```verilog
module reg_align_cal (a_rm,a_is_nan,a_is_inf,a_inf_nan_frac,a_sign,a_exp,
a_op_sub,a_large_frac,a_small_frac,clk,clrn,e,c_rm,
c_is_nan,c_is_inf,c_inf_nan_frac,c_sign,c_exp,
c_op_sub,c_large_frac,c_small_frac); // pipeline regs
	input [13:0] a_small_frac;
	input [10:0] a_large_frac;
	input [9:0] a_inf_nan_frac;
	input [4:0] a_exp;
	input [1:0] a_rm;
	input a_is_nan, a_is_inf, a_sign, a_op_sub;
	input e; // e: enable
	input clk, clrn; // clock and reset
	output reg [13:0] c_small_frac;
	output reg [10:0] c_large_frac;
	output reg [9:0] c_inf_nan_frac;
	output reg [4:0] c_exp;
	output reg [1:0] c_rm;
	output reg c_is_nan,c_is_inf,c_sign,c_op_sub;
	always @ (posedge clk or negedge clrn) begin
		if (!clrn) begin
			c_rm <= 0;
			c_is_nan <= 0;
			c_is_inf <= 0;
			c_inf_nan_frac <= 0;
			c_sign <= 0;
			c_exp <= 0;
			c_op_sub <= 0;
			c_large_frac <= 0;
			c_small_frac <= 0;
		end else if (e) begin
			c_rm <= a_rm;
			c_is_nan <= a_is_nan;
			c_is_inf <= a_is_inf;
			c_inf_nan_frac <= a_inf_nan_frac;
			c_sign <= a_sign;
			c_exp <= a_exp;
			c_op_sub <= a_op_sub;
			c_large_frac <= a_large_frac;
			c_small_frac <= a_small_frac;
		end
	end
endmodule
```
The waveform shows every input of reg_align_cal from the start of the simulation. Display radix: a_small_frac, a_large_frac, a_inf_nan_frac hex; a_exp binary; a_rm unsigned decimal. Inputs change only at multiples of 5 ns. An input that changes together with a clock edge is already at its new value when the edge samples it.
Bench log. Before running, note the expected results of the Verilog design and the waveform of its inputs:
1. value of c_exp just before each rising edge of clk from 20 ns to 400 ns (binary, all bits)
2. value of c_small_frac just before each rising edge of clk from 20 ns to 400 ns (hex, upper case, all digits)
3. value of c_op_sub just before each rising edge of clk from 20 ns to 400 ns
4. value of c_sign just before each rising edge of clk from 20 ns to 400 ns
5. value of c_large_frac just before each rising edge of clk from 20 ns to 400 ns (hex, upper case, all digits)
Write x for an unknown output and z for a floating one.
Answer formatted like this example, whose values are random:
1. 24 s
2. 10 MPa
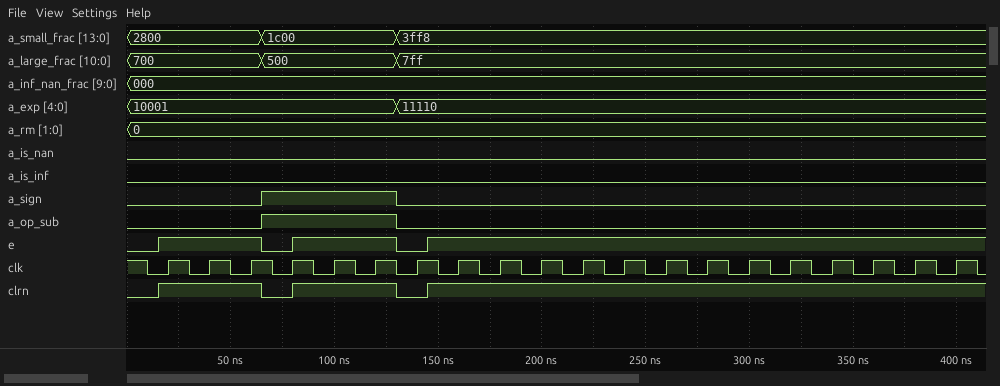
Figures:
1. 00000, 10001, 10001, 00000, 10001, 10001, 00000, 00000, 11110, 11110, 11110, 11110, 11110, 11110, 11110, 11110, 11110, 11110, 11110, 11110
2. 0000, 2800, 2800, 0000, 1C00, 1C00, 0000, 0000, 3FF8, 3FF8, 3FF8, 3FF8, 3FF8, 3FF8, 3FF8, 3FF8, 3FF8, 3FF8, 3FF8, 3FF8
3. 0 0 0 0 1 1 0 0 0 0 0 0 0 0 0 0 0 0 0 0
4. 0 0 0 0 1 1 0 0 0 0 0 0 0 0 0 0 0 0 0 0
5. 000, 700, 700, 000, 500, 500, 000, 000, 7FF, 7FF, 7FF, 7FF, 7FF, 7FF, 7FF, 7FF, 7FF, 7FF, 7FF, 7FF
